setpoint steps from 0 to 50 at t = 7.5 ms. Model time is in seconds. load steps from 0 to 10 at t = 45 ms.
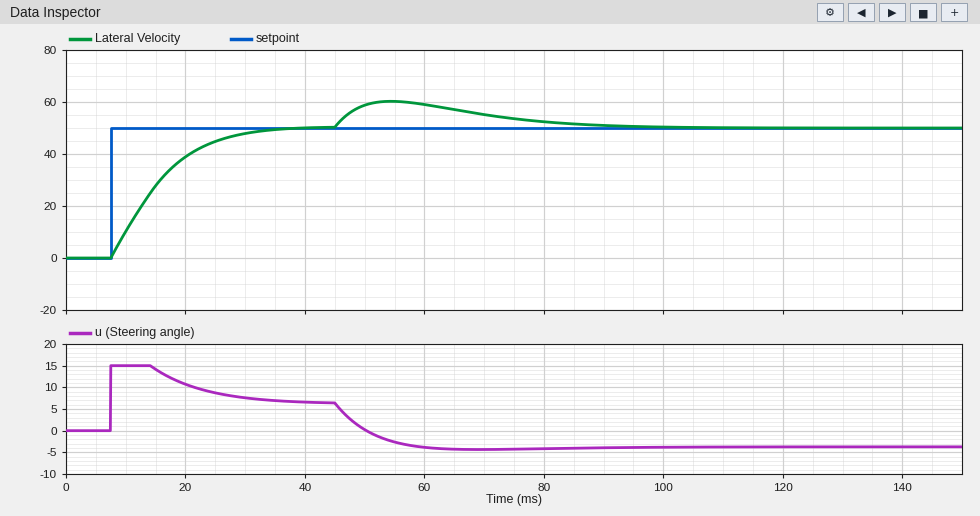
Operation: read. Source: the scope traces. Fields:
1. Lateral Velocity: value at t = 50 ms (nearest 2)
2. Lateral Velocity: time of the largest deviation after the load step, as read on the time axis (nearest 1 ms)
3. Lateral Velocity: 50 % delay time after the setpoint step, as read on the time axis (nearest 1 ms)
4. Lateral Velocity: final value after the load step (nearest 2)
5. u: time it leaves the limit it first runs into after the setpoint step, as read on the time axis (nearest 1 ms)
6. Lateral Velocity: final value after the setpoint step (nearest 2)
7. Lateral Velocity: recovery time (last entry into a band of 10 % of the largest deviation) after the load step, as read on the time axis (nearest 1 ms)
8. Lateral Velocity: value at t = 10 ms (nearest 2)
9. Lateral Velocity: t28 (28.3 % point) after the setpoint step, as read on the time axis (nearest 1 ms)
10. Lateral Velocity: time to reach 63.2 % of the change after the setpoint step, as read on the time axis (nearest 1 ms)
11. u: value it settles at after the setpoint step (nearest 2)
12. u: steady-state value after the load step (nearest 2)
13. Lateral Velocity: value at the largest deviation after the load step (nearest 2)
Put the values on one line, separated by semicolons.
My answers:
58; 54 ms; 14 ms; 50; 14 ms; 50; 90 ms; 10; 11 ms; 16 ms; 6; -4; 60
